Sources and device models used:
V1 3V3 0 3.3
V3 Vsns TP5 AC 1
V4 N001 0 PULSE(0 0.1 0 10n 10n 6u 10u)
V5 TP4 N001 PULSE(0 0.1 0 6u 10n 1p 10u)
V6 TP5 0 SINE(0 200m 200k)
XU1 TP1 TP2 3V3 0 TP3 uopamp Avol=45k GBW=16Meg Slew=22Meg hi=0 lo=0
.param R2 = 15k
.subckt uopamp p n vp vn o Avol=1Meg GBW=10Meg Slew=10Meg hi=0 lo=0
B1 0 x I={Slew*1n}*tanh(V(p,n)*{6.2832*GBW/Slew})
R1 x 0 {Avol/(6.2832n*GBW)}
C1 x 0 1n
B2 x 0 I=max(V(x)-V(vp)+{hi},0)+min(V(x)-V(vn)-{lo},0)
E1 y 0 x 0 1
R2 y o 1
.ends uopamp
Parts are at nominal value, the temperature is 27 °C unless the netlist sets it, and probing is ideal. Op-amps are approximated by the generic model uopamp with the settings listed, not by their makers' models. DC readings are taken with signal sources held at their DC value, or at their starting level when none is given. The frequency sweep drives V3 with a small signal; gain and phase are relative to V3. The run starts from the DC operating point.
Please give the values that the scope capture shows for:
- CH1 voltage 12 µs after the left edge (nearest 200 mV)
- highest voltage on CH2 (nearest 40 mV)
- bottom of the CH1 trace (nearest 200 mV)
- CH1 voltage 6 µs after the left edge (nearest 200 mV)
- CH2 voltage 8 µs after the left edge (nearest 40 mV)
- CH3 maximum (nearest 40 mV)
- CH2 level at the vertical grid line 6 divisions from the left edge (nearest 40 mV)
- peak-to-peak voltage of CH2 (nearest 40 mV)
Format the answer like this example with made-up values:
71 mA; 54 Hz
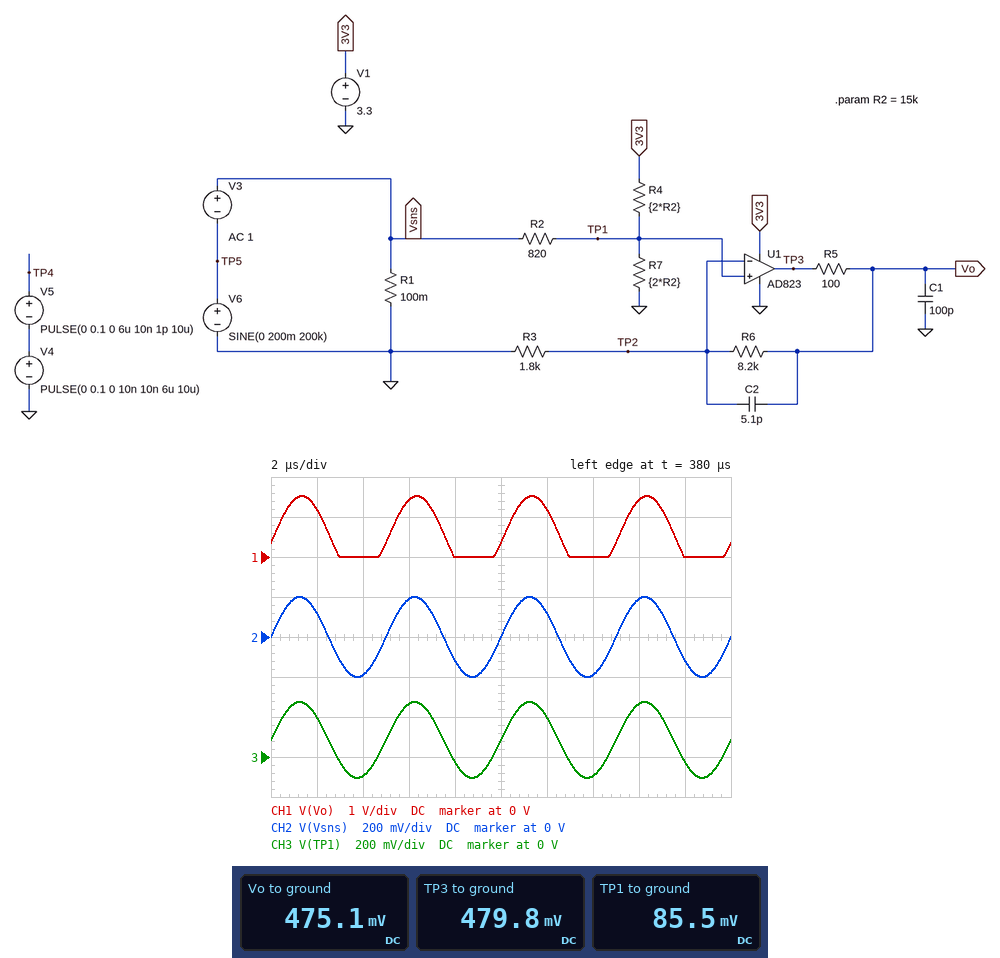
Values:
1.2 V; 200 mV; 0 V; 1.4 V; -120 mV; 280 mV; 120 mV; 400 mV
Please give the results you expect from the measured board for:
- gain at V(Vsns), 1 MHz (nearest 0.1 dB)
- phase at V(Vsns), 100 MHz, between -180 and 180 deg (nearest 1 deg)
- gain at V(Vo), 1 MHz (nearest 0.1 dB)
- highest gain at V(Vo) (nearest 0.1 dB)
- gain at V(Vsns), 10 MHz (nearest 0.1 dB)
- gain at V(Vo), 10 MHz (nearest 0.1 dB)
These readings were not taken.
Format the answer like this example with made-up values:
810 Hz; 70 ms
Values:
0 dB; 0 deg; 13.3 dB; 14.4 dB; 0 dB; -0.1 dB
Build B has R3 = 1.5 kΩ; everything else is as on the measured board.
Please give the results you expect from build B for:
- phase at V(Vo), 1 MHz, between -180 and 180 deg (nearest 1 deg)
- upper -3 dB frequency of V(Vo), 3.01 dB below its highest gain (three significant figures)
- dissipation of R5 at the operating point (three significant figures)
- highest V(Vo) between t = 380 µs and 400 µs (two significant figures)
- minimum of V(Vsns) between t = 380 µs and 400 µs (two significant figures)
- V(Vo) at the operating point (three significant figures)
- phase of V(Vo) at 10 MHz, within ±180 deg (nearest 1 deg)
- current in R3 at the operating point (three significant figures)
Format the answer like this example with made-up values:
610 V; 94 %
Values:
-33 deg; 1.66 MHz; 325 nW; 1.8 V; -200 mV; 553 mV; -98 deg; 57.0 µA
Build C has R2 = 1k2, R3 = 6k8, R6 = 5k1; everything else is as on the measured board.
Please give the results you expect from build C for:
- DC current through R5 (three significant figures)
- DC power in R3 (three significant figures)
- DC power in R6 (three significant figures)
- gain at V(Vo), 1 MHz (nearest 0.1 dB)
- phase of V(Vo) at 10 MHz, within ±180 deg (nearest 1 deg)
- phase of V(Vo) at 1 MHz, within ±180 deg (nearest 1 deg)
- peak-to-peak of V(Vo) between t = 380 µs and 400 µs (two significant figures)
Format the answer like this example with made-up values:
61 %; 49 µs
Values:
18.0 µA; 2.20 µW; 1.65 µW; 4.1 dB; -66 deg; -10 deg; 540 mV
